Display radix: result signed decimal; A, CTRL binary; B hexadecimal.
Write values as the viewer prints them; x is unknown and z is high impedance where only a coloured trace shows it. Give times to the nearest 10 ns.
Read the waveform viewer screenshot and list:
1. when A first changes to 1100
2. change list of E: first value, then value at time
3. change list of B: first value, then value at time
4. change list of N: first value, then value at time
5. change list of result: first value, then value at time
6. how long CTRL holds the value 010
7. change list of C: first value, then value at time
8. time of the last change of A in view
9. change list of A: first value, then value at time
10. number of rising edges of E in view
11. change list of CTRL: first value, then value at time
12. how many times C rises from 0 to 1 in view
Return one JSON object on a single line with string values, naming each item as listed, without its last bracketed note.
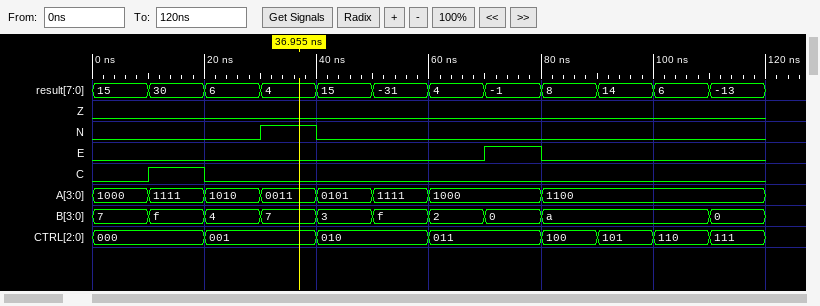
{"when A first changes to 1100": "80 ns", "change list of E: first value, then value at time": "0, 1 at 70 ns, 0 at 80 ns", "change list of B: first value, then value at time": "7, f at 10 ns, 4 at 20 ns, 7 at 30 ns, 3 at 40 ns, f at 50 ns, 2 at 60 ns, 0 at 70 ns, a at 80 ns, 0 at 110 ns", "change list of N: first value, then value at time": "0, 1 at 30 ns, 0 at 40 ns", "change list of result: first value, then value at time": "15, 30 at 10 ns, 6 at 20 ns, 4 at 30 ns, 15 at 40 ns, -31 at 50 ns, 4 at 60 ns, -1 at 70 ns, 8 at 80 ns, 14 at 90 ns, 6 at 100 ns, -13 at 110 ns", "how long CTRL holds the value 010": "20 ns", "change list of C: first value, then value at time": "0, 1 at 10 ns, 0 at 20 ns", "time of the last change of A in view": "80 ns", "change list of A: first value, then value at time": "1000, 1111 at 10 ns, 1010 at 20 ns, 0011 at 30 ns, 0101 at 40 ns, 1111 at 50 ns, 1000 at 60 ns, 1100 at 80 ns", "number of rising edges of E in view": "1", "change list of CTRL: first value, then value at time": "000, 001 at 20 ns, 010 at 40 ns, 011 at 60 ns, 100 at 80 ns, 101 at 90 ns, 110 at 100 ns, 111 at 110 ns", "how many times C rises from 0 to 1 in view": "1"}
